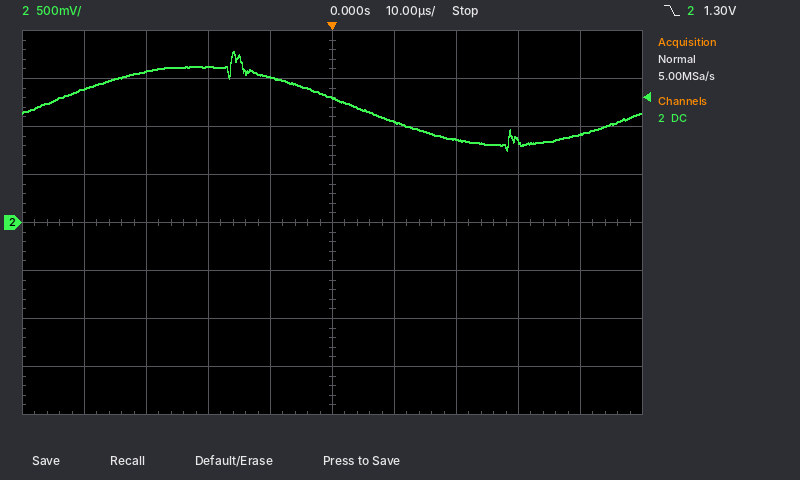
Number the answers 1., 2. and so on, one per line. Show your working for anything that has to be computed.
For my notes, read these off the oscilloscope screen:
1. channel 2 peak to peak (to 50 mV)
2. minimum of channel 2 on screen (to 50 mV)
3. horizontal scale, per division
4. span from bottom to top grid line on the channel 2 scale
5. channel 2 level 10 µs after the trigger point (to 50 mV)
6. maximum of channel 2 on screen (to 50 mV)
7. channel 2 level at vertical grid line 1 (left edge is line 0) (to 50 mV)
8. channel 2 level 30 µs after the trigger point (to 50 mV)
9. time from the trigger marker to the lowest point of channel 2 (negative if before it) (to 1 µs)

1. 1.80 V − (750 mV) = 1.05 V
2. 750 mV
3. 10 µs
4. 4 V
5. 1.05 V
6. 1.80 V
7. 1.40 V
8. 850 mV
9. +28 µs
